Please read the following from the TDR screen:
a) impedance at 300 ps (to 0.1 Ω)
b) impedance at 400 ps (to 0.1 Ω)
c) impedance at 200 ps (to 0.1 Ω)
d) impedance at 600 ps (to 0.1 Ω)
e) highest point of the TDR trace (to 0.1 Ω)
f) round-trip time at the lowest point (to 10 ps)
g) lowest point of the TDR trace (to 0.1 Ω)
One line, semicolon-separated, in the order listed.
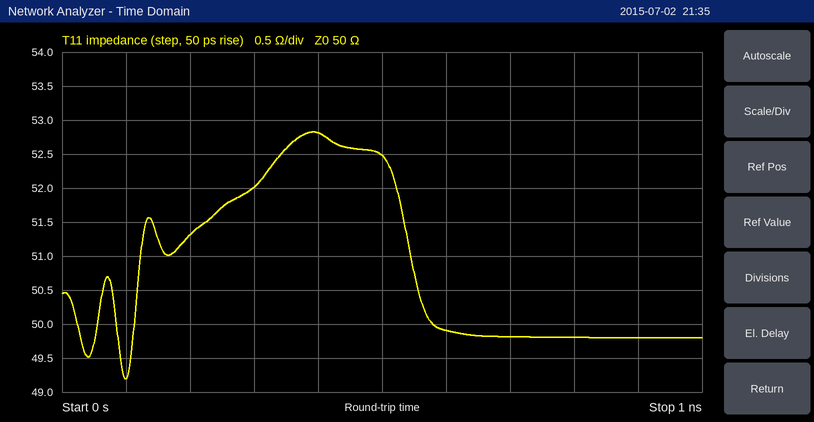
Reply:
52.0 Ω; 52.8 Ω; 51.3 Ω; 49.9 Ω; 52.8 Ω; 100 ps; 49.2 Ω
